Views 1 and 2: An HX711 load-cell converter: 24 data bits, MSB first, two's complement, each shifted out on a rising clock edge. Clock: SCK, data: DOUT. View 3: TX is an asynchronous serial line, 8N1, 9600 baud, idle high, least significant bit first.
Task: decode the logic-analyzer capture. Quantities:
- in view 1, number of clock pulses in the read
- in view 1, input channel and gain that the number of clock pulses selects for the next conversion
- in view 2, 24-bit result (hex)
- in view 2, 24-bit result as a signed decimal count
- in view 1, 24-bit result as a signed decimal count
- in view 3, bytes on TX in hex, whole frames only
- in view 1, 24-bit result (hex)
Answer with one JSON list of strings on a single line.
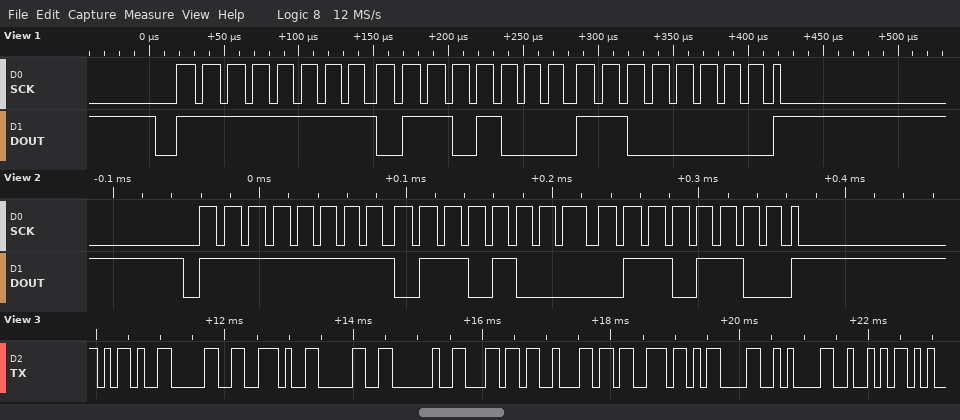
["25", "channel A, gain 128", "0xFF686C", "-38804", "-38720", "2D 30 2E 30 20 6C 62 73 0D 0A 52", "0xFF68C0"]
